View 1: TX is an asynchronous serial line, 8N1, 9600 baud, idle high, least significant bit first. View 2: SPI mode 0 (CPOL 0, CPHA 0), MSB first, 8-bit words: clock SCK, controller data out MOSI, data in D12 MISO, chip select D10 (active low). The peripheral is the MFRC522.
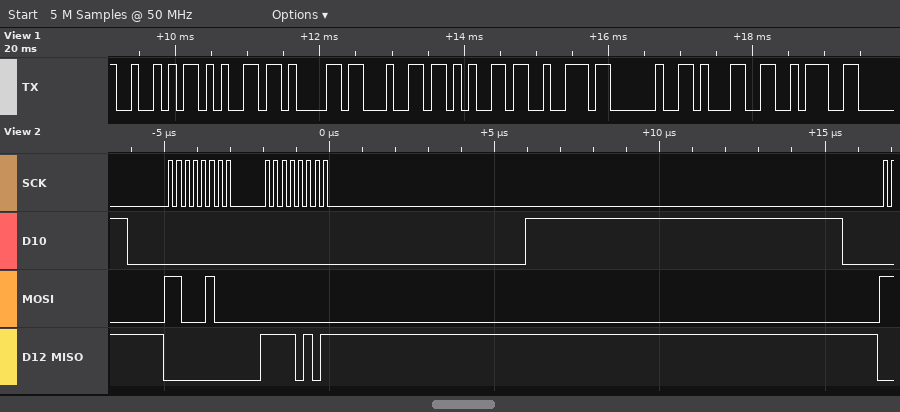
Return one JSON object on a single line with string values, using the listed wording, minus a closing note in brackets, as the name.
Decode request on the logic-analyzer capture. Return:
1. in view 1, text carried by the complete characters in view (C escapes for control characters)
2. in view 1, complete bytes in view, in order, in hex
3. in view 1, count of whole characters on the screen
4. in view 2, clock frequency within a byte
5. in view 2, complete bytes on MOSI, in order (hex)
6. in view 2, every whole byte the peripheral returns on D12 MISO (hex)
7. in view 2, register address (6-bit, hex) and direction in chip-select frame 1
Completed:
{"in view 1, text carried by the complete characters in view": "\"Reader 1:\"", "in view 1, complete bytes in view, in order, in hex": "52 65 61 64 65 72 20 31 3A", "in view 1, count of whole characters on the screen": "9", "in view 2, clock frequency within a byte": "4 MHz", "in view 2, complete bytes on MOSI, in order": "C4 00", "in view 2, every whole byte the peripheral returns on D12 MISO": "00 F5", "in view 2, register address (6-bit, hex) and direction in chip-select frame 1": "0x22 read"}
